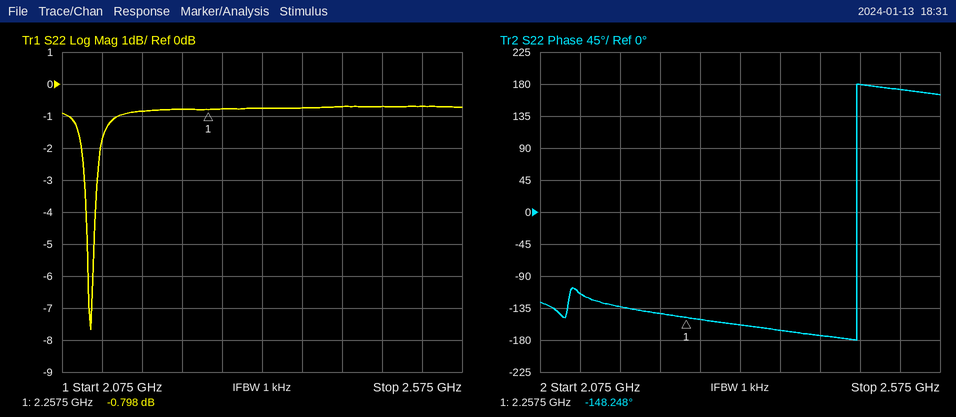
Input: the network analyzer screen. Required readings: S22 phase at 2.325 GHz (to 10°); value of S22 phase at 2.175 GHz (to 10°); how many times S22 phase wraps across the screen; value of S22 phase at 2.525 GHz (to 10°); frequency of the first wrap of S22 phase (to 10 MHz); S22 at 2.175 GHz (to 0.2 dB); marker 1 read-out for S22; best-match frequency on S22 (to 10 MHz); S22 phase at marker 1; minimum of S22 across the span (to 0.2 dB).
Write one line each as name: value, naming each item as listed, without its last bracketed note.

S22 phase at 2.325 GHz: -160°
value of S22 phase at 2.175 GHz: -130°
how many times S22 phase wraps across the screen: 1
value of S22 phase at 2.525 GHz: 170°
frequency of the first wrap of S22 phase: 2.47 GHz
S22 at 2.175 GHz: -0.8 dB
marker 1 read-out for S22: -0.798 dB
best-match frequency on S22: 2.11 GHz
S22 phase at marker 1: -148.248°
minimum of S22 across the span: -7.6 dB
